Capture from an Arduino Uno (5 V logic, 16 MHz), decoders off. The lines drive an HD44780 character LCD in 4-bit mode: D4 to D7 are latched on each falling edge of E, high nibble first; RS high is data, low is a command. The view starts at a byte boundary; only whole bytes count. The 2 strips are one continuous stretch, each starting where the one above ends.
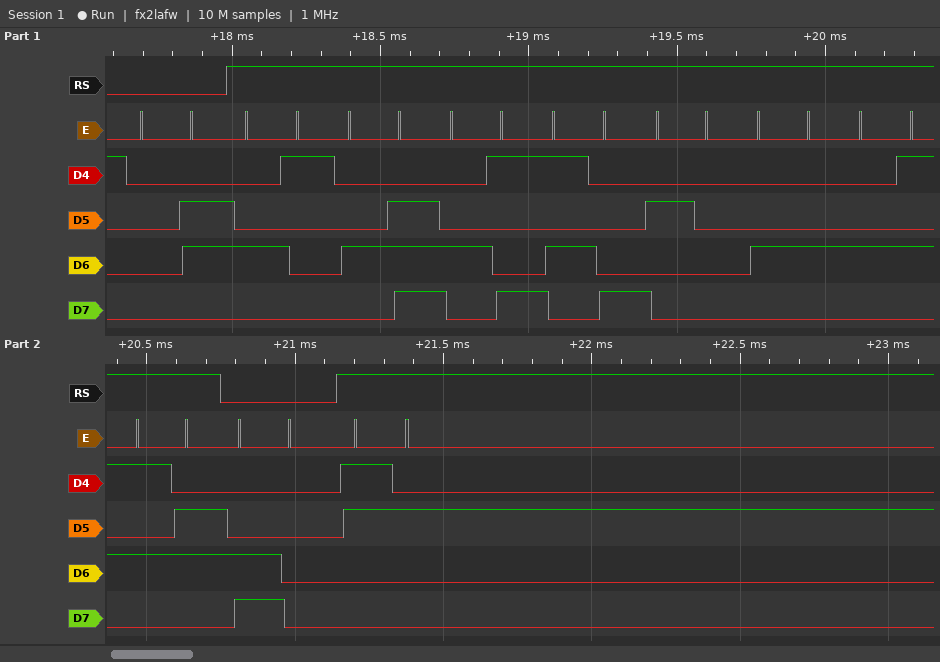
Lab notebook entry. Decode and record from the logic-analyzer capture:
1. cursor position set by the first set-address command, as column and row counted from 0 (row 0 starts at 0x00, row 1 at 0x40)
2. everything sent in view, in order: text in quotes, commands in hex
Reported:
column 0, row 1
0x06 "ANIX DEV" 0xC0 "2"
